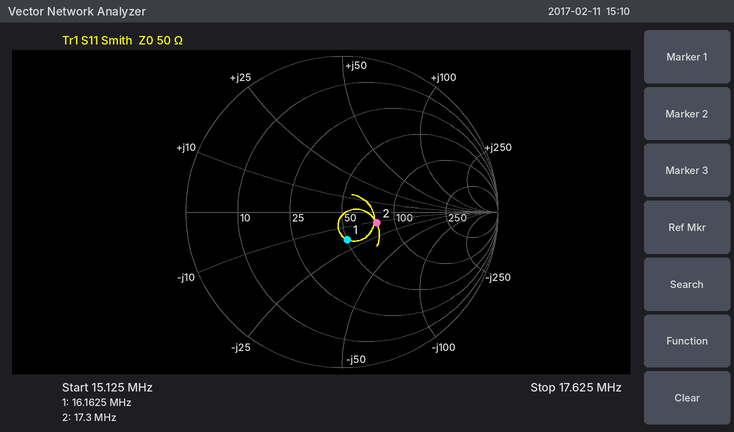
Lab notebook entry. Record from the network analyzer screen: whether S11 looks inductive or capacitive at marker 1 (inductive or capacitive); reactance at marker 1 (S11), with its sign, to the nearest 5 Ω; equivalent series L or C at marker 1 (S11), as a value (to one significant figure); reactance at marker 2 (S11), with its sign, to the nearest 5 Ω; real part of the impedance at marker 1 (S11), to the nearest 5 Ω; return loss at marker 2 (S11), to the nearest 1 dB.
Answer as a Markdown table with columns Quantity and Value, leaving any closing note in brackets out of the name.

| Quantity | Value |
|---|---|
| whether S11 looks inductive or capacitive at marker 1 | capacitive |
| reactance at marker 1 (S11), with its sign, to the nearest 5 Ω | -20 Ω |
| equivalent series L or C at marker 1 (S11), as a value | 500 pF |
| reactance at marker 2 (S11), with its sign, to the nearest 5 Ω | -10 Ω |
| real part of the impedance at marker 1 (S11), to the nearest 5 Ω | 50 Ω |
| return loss at marker 2 (S11), to the nearest 1 dB | 13 dB |
